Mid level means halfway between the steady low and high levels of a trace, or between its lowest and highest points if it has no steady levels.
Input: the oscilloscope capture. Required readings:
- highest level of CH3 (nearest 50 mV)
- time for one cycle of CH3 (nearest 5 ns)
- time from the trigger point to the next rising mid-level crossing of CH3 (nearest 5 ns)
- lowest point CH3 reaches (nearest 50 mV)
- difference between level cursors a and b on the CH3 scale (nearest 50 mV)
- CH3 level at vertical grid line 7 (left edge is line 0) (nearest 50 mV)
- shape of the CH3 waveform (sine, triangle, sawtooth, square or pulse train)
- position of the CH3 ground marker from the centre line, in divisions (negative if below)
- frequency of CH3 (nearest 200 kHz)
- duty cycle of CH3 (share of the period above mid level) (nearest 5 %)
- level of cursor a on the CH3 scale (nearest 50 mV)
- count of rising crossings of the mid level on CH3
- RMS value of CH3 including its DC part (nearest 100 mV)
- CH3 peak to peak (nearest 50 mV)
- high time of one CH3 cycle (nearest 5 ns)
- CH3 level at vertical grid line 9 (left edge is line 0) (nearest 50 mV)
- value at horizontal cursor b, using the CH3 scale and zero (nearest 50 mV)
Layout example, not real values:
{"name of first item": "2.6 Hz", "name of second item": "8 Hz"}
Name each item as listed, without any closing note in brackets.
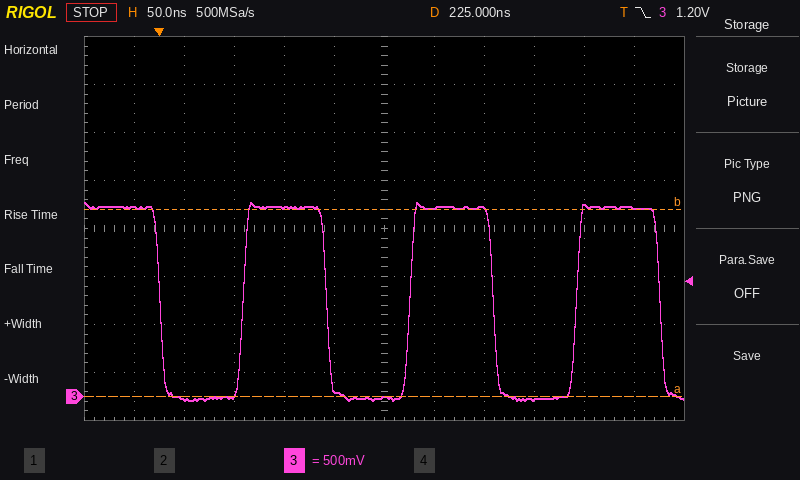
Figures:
{"highest level of CH3": "2.00 V", "time for one cycle of CH3": "165 ns", "time from the trigger point to the next rising mid-level crossing of CH3": "85 ns", "lowest point CH3 reaches": "-50 mV", "difference between level cursors a and b on the CH3 scale": "1.95 V", "CH3 level at vertical grid line 7 (left edge is line 0)": "1.95 V", "shape of the CH3 waveform": "square", "position of the CH3 ground marker from the centre line, in divisions": "-3.5 div", "frequency of CH3": "6.0 MHz", "duty cycle of CH3 (share of the period above mid level)": "50 %", "level of cursor a on the CH3 scale": "0 mV", "count of rising crossings of the mid level on CH3": "3", "RMS value of CH3 including its DC part": "1.4 V", "CH3 peak to peak": "2.05 V", "high time of one CH3 cycle": "85 ns", "CH3 level at vertical grid line 9 (left edge is line 0)": "-50 mV", "value at horizontal cursor b, using the CH3 scale and zero": "1.95 V"}
